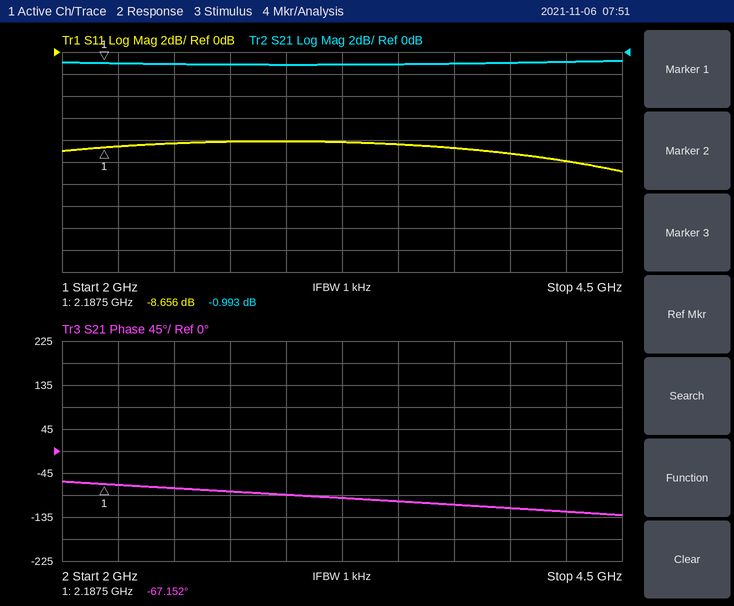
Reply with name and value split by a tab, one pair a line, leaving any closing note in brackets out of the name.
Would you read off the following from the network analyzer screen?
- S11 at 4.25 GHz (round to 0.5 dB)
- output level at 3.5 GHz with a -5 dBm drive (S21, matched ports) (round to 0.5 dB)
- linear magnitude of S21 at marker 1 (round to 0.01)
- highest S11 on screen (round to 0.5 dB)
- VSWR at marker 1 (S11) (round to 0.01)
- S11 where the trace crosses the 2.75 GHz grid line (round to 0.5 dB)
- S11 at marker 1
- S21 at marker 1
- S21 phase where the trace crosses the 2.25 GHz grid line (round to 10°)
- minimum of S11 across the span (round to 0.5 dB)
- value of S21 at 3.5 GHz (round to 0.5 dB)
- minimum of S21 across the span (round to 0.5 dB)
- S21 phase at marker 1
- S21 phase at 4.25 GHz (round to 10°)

S11 at 4.25 GHz	-10.0 dB
output level at 3.5 GHz with a -5 dBm drive (S21, matched ports)	-6.0 dBm
linear magnitude of S21 at marker 1	0.89
highest S11 on screen	-8.0 dB
VSWR at marker 1 (S11)	2.17
S11 where the trace crosses the 2.75 GHz grid line	-8.0 dB
S11 at marker 1	-8.656 dB
S21 at marker 1	-0.993 dB
S21 phase where the trace crosses the 2.25 GHz grid line	-70°
minimum of S11 across the span	-11.0 dB
value of S21 at 3.5 GHz	-1.0 dB
minimum of S21 across the span	-1.0 dB
S21 phase at marker 1	-67.152°
S21 phase at 4.25 GHz	-120°
